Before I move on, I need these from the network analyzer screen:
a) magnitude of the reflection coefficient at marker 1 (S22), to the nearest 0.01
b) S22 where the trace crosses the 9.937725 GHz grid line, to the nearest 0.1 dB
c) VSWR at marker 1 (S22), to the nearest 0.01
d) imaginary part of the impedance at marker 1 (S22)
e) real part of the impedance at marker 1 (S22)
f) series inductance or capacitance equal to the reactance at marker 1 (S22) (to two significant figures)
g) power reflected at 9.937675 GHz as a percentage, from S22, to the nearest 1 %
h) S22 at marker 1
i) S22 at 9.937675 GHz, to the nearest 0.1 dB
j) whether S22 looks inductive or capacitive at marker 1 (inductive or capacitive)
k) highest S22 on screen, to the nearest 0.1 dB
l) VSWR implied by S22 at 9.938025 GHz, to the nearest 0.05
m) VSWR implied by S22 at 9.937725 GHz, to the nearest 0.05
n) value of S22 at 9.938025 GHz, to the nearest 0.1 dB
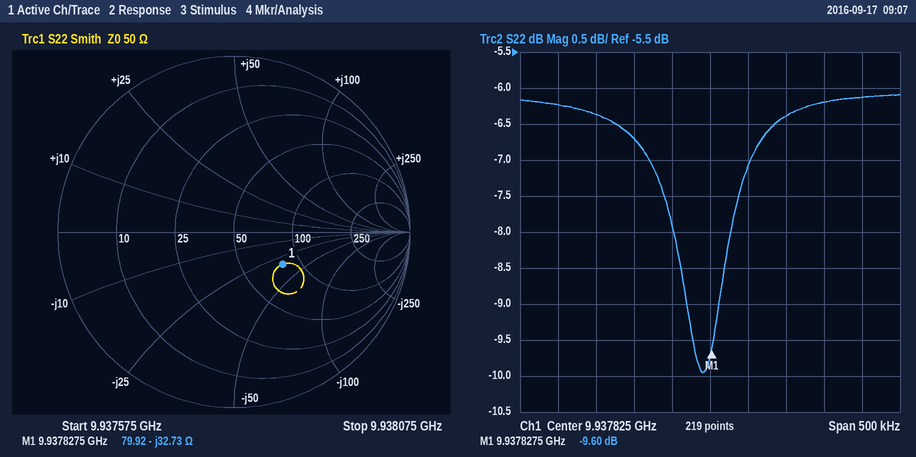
0.33
-6.7 dB
1.99
-32.73 Ω
79.92 Ω
490 fF
23 %
-9.60 dB
-6.4 dB
capacitive
-6.1 dB
2.95
2.70
-6.1 dB
